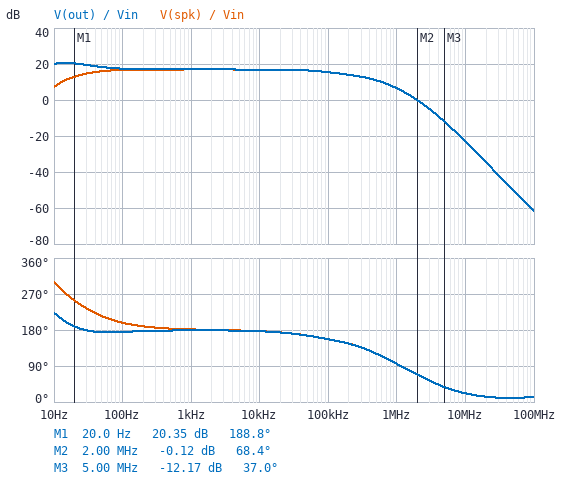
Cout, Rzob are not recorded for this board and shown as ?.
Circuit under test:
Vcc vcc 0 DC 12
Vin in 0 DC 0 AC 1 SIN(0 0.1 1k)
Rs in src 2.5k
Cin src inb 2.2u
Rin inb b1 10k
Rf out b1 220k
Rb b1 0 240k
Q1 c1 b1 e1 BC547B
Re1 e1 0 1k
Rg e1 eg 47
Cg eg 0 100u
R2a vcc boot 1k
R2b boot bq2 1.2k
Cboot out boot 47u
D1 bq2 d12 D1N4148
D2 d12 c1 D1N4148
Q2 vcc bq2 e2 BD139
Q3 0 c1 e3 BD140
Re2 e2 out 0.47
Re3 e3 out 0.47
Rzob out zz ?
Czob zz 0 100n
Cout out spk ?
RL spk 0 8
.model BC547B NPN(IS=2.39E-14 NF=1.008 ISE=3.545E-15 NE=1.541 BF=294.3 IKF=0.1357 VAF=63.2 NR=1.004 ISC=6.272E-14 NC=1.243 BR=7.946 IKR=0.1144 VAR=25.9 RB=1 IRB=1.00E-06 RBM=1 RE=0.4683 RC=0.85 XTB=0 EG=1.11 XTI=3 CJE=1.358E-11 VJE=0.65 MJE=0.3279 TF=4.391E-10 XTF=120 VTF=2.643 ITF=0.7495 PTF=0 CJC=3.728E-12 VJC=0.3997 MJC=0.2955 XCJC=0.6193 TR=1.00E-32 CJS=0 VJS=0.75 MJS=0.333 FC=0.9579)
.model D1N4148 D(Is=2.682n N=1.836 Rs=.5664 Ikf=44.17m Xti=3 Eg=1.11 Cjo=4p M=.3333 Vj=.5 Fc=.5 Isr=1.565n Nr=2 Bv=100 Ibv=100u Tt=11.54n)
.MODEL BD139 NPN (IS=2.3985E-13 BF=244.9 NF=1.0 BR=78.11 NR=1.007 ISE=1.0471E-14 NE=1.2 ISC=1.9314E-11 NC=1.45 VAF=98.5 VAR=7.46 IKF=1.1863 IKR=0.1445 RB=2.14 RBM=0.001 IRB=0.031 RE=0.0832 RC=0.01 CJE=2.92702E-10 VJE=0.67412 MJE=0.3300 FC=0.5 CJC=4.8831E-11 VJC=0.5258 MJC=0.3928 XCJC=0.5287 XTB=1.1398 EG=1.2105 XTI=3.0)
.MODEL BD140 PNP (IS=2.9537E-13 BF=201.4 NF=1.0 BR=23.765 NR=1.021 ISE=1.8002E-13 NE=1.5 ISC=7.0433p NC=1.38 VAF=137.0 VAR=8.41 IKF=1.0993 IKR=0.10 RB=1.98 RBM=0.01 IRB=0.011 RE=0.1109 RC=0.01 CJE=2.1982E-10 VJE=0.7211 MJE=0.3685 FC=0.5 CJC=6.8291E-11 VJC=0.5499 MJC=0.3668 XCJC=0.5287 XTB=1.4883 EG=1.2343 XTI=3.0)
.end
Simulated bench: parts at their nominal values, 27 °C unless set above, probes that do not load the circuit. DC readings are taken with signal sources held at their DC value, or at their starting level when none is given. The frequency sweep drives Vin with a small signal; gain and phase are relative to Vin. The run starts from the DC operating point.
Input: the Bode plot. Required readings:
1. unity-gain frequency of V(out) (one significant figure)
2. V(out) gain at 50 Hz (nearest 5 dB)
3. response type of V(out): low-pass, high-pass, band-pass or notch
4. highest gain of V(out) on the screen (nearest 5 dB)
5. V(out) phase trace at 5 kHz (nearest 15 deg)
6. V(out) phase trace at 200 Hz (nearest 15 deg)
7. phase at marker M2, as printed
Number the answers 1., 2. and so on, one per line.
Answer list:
1. 2 MHz
2. 20 dB
3. low-pass
4. 20 dB
5. 180 deg
6. 180 deg
7. 68.4 deg
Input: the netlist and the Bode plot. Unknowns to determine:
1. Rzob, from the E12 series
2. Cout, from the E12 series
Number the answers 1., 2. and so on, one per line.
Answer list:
1. 12 Ω
2. 470 µF
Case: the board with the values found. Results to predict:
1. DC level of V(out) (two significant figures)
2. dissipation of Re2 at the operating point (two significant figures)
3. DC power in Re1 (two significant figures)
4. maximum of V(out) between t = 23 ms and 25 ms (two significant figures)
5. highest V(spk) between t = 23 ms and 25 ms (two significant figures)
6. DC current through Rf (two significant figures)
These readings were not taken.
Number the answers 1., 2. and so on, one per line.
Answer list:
1. 6.8 V
2. 92 µW
3. 4.3 mW
4. 7.5 V
5. 700 mV
6. 18 µA
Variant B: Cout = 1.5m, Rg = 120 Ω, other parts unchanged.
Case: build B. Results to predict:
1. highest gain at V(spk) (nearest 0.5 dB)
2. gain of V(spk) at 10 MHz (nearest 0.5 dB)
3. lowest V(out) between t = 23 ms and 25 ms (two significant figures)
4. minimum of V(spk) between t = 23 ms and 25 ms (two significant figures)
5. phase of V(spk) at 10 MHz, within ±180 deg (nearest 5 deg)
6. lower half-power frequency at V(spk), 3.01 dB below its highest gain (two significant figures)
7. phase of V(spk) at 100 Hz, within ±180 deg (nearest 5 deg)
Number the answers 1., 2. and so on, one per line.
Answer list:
1. 14.0 dB
2. -24.0 dB
3. 6.3 V
4. -500 mV
5. 25 deg
6. 11 Hz
7. -170 deg
